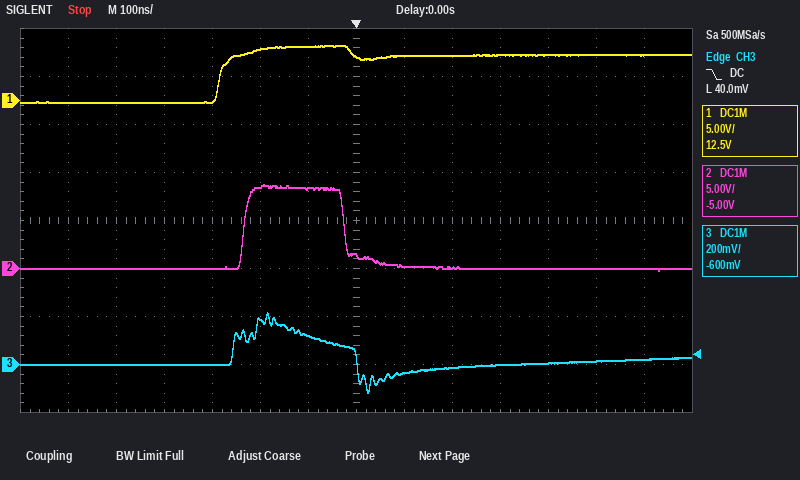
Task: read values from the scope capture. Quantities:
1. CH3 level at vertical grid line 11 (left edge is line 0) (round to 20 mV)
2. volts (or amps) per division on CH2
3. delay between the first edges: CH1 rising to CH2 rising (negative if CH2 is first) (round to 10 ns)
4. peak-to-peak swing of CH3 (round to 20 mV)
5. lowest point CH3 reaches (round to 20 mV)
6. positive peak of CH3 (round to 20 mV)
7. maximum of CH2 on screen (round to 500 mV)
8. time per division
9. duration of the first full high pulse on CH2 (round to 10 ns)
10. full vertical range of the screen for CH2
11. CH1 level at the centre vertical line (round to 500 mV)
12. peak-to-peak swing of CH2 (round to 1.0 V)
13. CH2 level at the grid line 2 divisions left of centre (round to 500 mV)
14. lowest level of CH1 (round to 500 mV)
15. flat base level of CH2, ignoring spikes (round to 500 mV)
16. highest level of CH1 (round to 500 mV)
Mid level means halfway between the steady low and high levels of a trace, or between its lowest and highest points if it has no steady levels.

0 mV
5 V
+50 ns
340 mV
-120 mV
220 mV
9.0 V
100 ns
210 ns
40 V
4.5 V
9.0 V
8.5 V
0.0 V
0.0 V
5.5 V
